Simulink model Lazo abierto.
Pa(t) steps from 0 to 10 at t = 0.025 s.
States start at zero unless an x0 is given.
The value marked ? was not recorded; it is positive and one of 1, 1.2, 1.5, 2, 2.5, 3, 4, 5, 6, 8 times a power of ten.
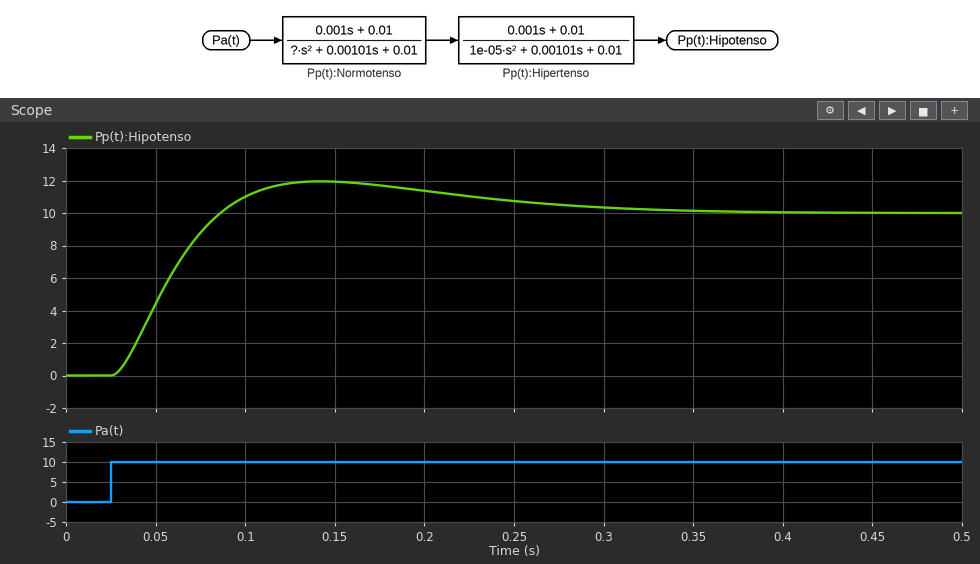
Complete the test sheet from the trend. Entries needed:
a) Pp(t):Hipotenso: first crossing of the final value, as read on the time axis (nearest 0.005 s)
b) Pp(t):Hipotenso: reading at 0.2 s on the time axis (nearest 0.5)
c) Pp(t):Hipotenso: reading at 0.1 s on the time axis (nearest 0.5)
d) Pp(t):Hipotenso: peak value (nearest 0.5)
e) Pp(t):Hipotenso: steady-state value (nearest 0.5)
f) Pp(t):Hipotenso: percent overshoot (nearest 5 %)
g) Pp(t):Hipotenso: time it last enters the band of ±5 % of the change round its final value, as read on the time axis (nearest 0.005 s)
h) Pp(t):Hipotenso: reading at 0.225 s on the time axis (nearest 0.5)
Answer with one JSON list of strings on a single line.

["0.085 s", "11.5", "11.0", "12.0", "10.0", "20 %", "0.275 s", "11.0"]
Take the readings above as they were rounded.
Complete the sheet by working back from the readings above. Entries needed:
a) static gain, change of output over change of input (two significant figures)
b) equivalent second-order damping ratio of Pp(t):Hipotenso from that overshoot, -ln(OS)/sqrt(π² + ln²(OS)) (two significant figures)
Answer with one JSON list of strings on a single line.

["1.0", "0.46"]
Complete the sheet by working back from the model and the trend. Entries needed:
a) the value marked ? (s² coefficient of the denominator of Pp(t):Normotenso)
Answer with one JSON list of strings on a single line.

["3e-05"]
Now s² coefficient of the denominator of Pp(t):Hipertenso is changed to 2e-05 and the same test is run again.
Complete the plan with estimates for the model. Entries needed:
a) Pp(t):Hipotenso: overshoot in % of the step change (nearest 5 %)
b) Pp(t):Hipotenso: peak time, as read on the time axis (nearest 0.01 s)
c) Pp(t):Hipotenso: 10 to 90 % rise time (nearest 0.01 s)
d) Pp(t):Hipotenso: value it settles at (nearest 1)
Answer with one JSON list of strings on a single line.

["25 %", "0.15 s", "0.05 s", "10"]
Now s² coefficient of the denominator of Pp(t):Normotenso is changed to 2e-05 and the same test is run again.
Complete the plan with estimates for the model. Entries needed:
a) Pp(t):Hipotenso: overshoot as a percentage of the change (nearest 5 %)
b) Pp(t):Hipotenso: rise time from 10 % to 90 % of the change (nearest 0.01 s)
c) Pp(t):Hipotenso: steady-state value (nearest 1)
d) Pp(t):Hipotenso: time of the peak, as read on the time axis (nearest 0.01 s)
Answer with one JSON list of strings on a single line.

["15 %", "0.03 s", "10", "0.12 s"]
